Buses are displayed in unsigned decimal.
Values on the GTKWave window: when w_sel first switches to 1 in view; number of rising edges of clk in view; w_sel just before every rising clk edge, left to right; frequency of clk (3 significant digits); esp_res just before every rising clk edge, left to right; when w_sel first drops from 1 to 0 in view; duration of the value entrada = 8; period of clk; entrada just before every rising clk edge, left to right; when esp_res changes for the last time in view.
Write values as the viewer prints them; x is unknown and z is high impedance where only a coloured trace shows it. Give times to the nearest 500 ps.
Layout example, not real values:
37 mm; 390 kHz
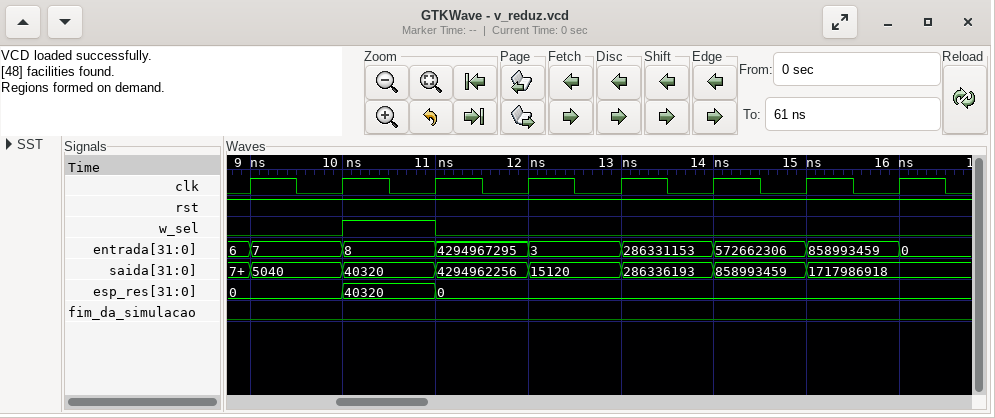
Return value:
10000 ps; 8; 0 0 1 0 0 0 0 0; 1.00 GHz; 0, 0, 40320, 0, 0, 0, 0, 0; 11000 ps; 1000 ps; 1000 ps; 6, 7, 8, 4294967295, 3, 286331153, 572662306, 858993459; 11000 ps
